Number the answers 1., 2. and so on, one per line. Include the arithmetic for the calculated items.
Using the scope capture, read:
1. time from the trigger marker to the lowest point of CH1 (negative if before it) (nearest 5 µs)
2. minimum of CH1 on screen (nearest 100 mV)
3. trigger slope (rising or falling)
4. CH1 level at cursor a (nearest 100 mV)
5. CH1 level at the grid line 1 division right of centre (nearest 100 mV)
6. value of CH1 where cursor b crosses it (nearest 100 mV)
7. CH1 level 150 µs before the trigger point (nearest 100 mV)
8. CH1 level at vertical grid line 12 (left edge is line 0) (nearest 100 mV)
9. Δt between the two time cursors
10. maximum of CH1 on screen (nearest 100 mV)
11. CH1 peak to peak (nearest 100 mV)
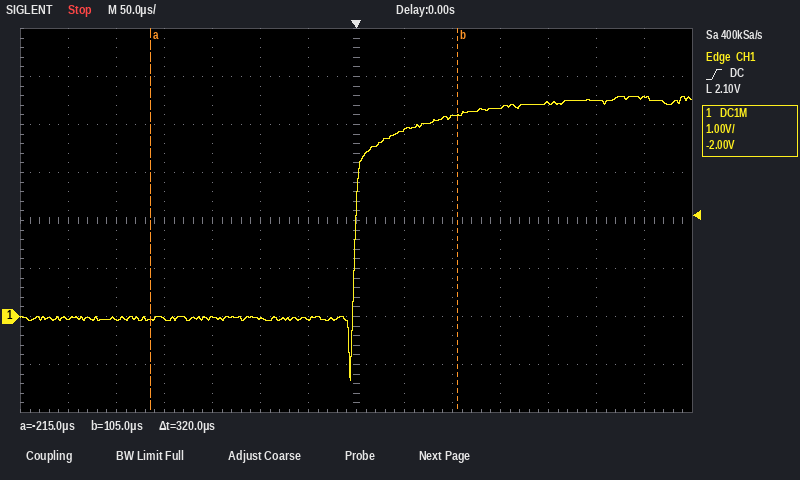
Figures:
1. -5 µs
2. -1.3 V
3. rising
4. -100 mV
5. 3.9 V
6. 4.2 V
7. 0.0 V
8. 4.5 V
9. 320 µs
10. 4.6 V
11. 4.6 V − (-1.3 V) = 5.9 V
